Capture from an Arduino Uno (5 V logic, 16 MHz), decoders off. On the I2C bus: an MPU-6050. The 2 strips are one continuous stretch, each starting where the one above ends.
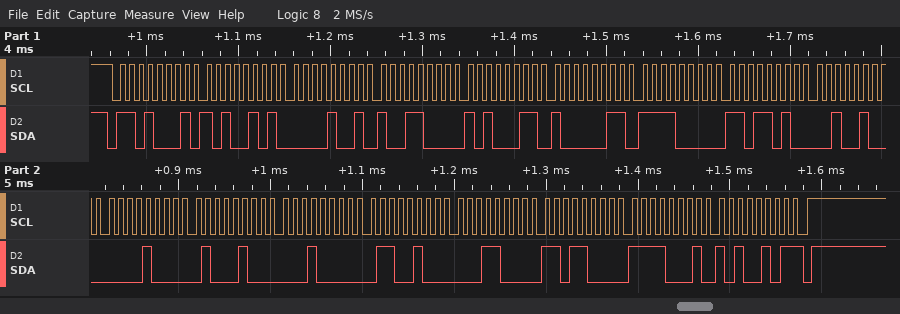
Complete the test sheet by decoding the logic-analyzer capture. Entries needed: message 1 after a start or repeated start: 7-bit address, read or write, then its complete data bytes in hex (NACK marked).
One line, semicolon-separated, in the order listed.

0x68 read: A5 09 98 A3 83 F0 DA 24 08 44 10 64 18 D8 F1 A5 NACK
